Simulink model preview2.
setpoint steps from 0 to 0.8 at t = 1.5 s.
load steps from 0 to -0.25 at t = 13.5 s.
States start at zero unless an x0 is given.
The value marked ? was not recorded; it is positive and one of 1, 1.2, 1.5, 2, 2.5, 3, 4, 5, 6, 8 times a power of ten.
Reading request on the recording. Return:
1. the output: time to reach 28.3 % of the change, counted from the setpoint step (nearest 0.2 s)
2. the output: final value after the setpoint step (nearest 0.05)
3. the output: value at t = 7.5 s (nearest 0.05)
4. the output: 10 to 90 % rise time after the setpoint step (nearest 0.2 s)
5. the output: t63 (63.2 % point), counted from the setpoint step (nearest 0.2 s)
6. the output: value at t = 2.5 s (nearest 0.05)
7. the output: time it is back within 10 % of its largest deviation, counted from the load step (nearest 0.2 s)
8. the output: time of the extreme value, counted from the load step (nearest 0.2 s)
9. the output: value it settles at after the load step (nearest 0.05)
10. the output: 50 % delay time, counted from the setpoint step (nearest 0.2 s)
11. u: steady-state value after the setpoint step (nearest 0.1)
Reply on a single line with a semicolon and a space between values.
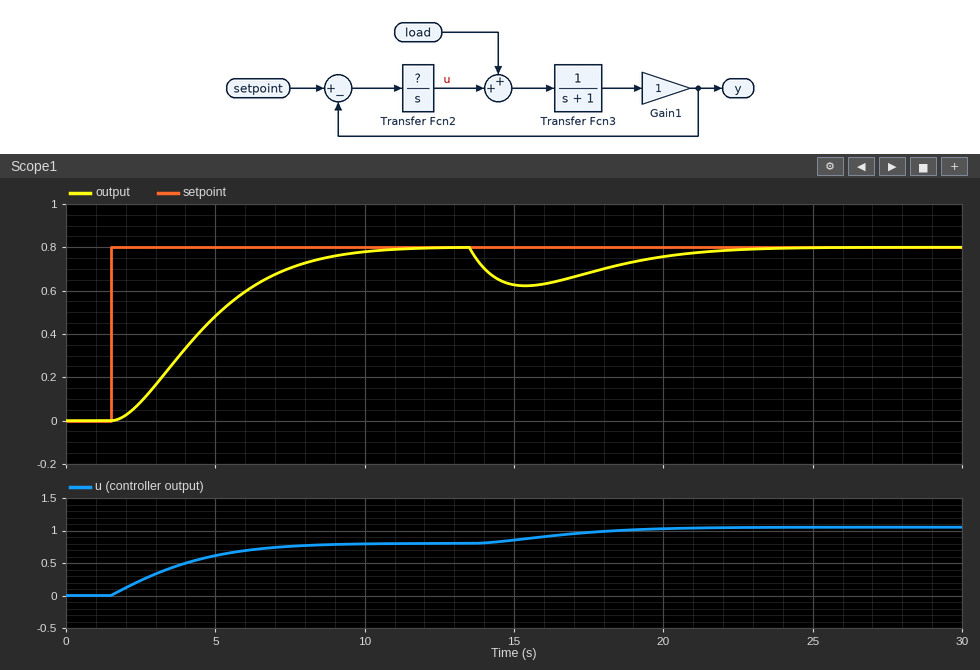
1.8 s; 0.80; 0.70; 5.4 s; 3.6 s; 0.10; 8.2 s; 1.8 s; 0.80; 3.0 s; 0.8
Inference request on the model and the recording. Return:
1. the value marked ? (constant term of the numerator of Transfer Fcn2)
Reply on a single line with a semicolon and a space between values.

0.3
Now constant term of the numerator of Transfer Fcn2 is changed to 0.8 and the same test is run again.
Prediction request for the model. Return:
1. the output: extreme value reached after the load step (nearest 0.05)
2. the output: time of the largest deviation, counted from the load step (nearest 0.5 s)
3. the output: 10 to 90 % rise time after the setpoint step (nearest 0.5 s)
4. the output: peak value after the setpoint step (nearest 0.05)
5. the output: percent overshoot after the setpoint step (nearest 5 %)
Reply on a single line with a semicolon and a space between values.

0.65; 1.5 s; 2.0 s; 0.90; 10 %
